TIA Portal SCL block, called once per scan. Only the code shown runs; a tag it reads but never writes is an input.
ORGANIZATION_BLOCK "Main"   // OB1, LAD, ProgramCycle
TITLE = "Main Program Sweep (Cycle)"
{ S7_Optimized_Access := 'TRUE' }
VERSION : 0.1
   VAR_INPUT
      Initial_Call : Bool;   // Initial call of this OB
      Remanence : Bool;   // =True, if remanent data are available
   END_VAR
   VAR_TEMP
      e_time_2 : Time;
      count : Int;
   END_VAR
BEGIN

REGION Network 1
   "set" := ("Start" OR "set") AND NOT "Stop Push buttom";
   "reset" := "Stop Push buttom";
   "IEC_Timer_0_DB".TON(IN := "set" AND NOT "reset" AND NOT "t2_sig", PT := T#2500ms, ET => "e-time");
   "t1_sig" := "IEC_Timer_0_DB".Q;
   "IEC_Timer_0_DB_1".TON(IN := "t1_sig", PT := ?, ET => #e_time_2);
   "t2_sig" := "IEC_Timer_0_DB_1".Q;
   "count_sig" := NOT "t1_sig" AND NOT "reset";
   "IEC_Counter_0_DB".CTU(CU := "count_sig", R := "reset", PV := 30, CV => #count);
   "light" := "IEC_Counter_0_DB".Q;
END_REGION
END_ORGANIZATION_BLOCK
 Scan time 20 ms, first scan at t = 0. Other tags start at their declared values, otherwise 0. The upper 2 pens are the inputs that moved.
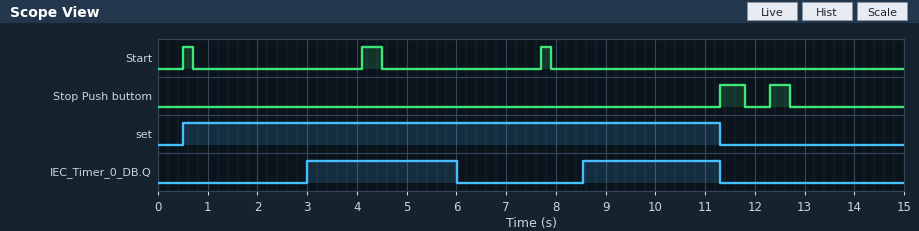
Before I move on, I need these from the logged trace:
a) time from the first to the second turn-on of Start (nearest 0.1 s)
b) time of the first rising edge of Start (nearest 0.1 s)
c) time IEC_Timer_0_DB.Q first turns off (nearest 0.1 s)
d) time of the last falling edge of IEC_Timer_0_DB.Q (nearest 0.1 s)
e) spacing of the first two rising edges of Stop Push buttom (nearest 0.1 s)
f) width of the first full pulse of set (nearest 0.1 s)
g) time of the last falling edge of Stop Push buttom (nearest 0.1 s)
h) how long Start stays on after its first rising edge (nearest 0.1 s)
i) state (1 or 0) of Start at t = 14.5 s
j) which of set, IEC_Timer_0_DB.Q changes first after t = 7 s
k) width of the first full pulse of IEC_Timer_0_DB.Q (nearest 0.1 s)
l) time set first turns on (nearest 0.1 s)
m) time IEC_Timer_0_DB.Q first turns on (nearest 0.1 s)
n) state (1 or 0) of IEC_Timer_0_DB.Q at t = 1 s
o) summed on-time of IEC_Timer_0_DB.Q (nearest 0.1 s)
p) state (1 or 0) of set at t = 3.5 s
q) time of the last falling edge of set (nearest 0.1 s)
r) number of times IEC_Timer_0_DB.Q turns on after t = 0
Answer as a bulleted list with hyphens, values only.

- 3.6 s
- 0.5 s
- 6.0 s
- 11.3 s
- 1.0 s
- 10.8 s
- 12.7 s
- 0.2 s
- 0
- IEC_Timer_0_DB.Q
- 3.0 s
- 0.5 s
- 3.0 s
- 0
- 5.8 s
- 1
- 11.3 s
- 2
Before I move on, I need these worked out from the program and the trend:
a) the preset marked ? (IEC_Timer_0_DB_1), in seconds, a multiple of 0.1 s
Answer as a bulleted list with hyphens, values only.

- 3.0 s
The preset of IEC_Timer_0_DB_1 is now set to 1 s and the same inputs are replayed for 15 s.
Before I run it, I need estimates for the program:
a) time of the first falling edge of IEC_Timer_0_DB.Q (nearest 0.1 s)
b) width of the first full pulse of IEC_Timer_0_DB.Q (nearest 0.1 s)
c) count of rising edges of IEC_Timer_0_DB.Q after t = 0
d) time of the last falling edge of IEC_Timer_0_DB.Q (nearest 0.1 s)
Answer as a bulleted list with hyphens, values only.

- 4.0 s
- 1.0 s
- 3
- 11.1 s
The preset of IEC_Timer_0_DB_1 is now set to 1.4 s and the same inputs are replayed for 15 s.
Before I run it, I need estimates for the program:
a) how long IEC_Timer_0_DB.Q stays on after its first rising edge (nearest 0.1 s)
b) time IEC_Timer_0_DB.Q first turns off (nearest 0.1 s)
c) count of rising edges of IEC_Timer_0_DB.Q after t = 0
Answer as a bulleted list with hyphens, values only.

- 1.4 s
- 4.4 s
- 3
